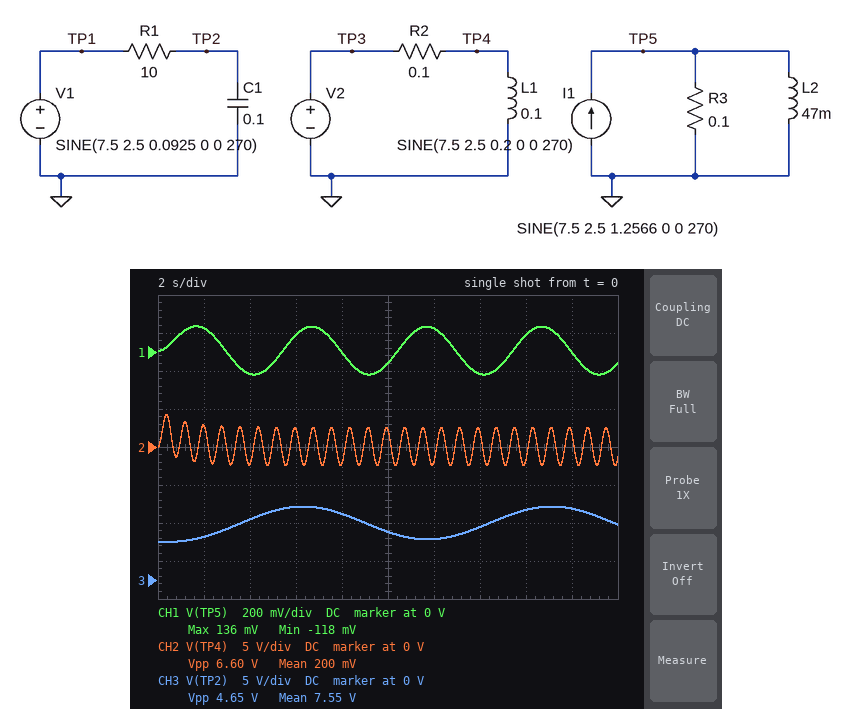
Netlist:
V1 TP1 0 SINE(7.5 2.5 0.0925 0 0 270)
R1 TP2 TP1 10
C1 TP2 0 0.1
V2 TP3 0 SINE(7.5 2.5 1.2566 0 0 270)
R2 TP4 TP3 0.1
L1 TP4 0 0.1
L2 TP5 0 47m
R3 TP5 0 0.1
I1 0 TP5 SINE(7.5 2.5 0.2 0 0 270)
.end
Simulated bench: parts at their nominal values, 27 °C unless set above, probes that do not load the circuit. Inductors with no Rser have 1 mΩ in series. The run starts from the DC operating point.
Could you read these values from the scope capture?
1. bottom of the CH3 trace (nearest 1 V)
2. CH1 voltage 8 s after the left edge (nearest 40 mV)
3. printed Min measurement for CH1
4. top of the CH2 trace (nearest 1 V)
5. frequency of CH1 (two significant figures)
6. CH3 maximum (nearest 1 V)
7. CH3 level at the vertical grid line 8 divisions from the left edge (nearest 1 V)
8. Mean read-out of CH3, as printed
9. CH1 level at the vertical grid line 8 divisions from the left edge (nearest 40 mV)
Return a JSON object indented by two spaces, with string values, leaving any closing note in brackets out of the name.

{
  "bottom of the CH3 trace": "5 V",
  "CH1 voltage 8 s after the left edge": "0 V",
  "printed Min measurement for CH1": "-118 mV",
  "top of the CH2 trace": "4 V",
  "frequency of CH1": "200 mHz",
  "CH3 maximum": "10 V",
  "CH3 level at the vertical grid line 8 divisions from the left edge": "9 V",
  "Mean read-out of CH3, as printed": "7.55 V",
  "CH1 level at the vertical grid line 8 divisions from the left edge": "80 mV"
}
